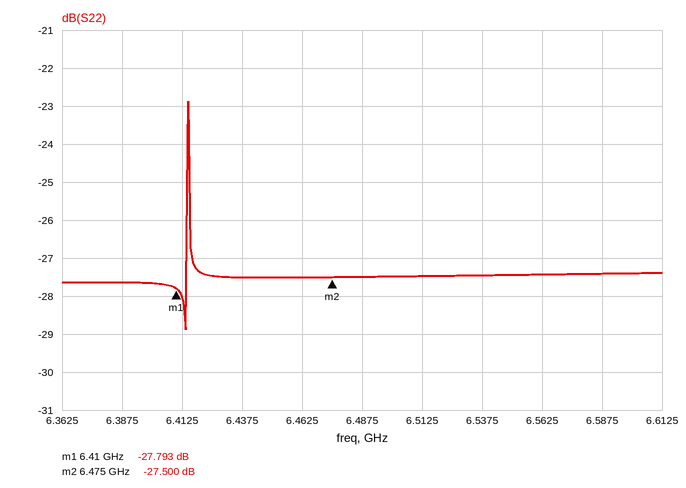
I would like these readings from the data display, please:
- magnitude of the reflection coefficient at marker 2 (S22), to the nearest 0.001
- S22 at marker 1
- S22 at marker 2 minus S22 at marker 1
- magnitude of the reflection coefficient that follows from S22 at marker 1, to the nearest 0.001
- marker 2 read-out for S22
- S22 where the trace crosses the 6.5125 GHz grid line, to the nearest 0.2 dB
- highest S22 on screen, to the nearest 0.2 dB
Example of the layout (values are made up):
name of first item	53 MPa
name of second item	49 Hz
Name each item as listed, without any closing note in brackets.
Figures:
magnitude of the reflection coefficient at marker 2 (S22), to the nearest 0.001	0.042
S22 at marker 1	-27.793 dB
S22 at marker 2 minus S22 at marker 1	0.293 dB
magnitude of the reflection coefficient that follows from S22 at marker 1, to the nearest 0.001	0.041
marker 2 read-out for S22	-27.500 dB
S22 where the trace crosses the 6.5125 GHz grid line, to the nearest 0.2 dB	-27.4 dB
highest S22 on screen, to the nearest 0.2 dB	-22.8 dB
